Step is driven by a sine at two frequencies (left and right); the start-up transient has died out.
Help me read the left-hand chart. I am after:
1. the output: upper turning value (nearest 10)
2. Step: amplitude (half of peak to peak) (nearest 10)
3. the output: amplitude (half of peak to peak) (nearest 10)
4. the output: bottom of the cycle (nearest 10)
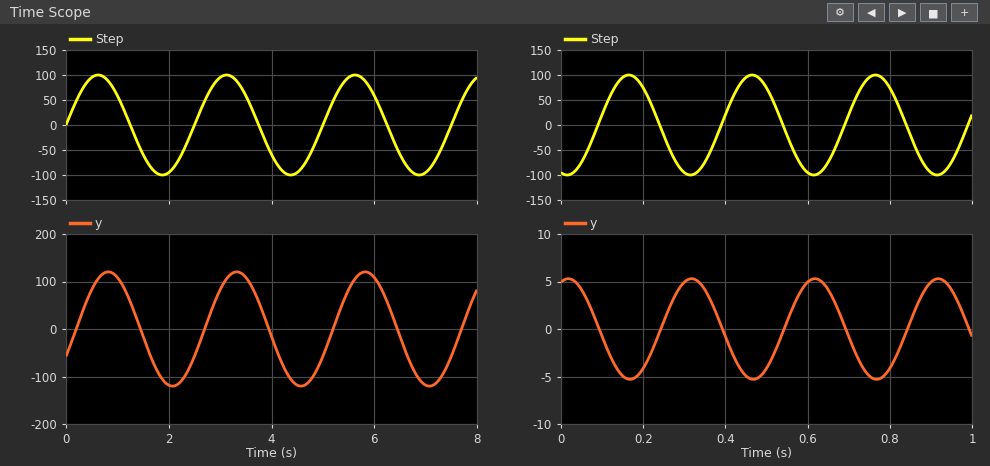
120
100
120
-120
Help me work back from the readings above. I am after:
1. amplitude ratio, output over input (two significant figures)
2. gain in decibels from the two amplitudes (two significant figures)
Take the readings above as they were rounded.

1.2
1.6 dB
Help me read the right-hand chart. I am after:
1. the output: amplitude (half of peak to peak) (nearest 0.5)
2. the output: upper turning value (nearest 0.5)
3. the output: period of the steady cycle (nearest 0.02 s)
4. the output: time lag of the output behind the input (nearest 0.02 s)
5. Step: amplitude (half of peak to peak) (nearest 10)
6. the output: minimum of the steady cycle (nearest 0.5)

5.5
5.5
0.30 s
0.16 s
100
-5.5
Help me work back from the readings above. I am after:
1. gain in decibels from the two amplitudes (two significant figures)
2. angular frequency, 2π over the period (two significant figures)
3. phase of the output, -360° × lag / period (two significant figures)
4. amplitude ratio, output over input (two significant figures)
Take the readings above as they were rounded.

-25 dB
21 rad/s
-190°
0.055
